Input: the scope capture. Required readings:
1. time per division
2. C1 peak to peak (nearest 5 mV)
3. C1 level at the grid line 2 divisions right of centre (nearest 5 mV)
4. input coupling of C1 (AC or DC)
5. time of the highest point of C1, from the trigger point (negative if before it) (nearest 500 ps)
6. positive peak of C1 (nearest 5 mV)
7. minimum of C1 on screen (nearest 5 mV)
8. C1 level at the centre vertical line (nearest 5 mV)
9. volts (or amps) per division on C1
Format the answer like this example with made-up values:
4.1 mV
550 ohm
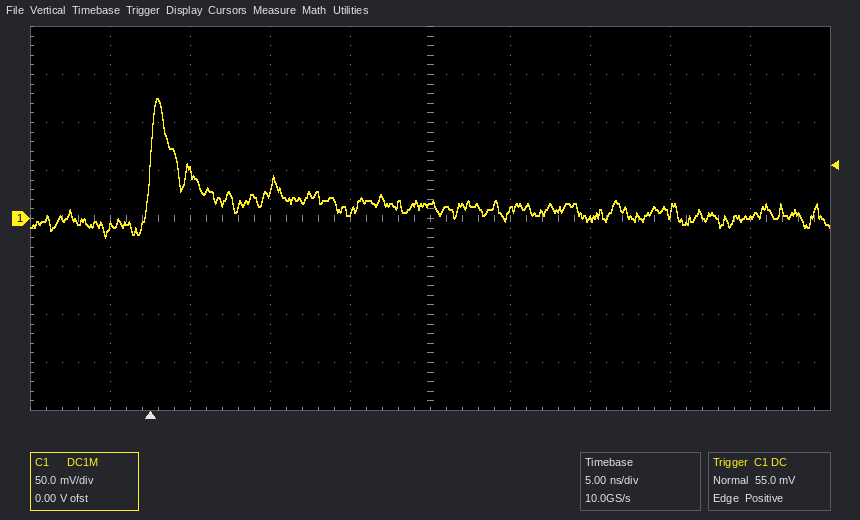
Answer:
5 ns
145 mV
0 mV
DC
+500 ps
125 mV
-20 mV
15 mV
50 mV
